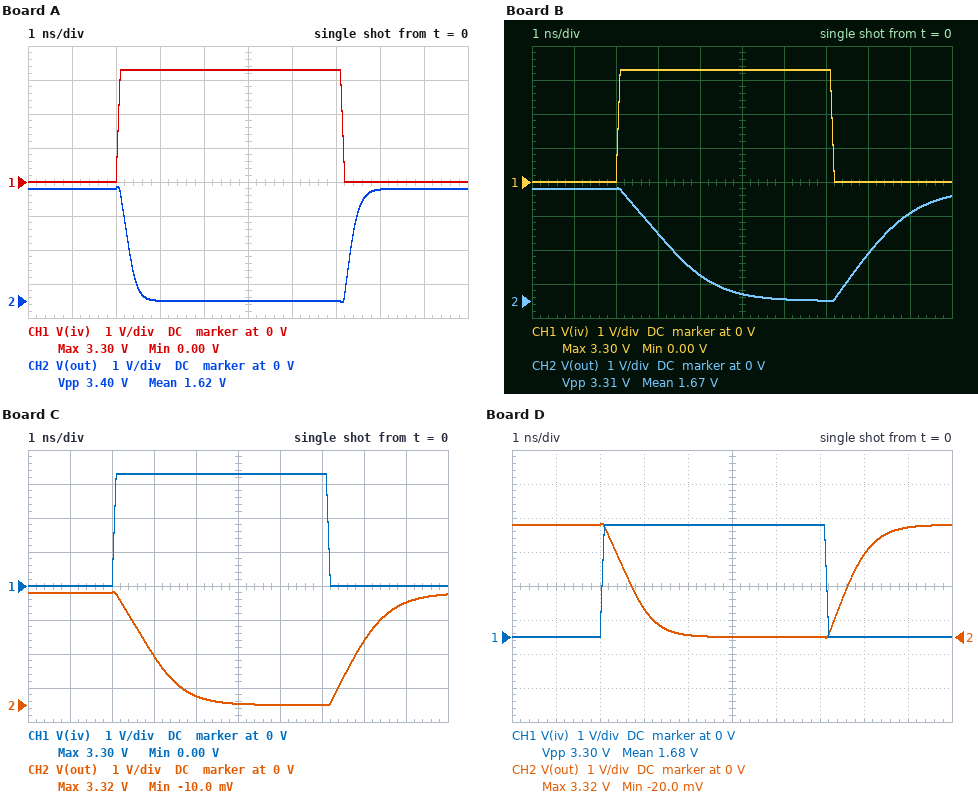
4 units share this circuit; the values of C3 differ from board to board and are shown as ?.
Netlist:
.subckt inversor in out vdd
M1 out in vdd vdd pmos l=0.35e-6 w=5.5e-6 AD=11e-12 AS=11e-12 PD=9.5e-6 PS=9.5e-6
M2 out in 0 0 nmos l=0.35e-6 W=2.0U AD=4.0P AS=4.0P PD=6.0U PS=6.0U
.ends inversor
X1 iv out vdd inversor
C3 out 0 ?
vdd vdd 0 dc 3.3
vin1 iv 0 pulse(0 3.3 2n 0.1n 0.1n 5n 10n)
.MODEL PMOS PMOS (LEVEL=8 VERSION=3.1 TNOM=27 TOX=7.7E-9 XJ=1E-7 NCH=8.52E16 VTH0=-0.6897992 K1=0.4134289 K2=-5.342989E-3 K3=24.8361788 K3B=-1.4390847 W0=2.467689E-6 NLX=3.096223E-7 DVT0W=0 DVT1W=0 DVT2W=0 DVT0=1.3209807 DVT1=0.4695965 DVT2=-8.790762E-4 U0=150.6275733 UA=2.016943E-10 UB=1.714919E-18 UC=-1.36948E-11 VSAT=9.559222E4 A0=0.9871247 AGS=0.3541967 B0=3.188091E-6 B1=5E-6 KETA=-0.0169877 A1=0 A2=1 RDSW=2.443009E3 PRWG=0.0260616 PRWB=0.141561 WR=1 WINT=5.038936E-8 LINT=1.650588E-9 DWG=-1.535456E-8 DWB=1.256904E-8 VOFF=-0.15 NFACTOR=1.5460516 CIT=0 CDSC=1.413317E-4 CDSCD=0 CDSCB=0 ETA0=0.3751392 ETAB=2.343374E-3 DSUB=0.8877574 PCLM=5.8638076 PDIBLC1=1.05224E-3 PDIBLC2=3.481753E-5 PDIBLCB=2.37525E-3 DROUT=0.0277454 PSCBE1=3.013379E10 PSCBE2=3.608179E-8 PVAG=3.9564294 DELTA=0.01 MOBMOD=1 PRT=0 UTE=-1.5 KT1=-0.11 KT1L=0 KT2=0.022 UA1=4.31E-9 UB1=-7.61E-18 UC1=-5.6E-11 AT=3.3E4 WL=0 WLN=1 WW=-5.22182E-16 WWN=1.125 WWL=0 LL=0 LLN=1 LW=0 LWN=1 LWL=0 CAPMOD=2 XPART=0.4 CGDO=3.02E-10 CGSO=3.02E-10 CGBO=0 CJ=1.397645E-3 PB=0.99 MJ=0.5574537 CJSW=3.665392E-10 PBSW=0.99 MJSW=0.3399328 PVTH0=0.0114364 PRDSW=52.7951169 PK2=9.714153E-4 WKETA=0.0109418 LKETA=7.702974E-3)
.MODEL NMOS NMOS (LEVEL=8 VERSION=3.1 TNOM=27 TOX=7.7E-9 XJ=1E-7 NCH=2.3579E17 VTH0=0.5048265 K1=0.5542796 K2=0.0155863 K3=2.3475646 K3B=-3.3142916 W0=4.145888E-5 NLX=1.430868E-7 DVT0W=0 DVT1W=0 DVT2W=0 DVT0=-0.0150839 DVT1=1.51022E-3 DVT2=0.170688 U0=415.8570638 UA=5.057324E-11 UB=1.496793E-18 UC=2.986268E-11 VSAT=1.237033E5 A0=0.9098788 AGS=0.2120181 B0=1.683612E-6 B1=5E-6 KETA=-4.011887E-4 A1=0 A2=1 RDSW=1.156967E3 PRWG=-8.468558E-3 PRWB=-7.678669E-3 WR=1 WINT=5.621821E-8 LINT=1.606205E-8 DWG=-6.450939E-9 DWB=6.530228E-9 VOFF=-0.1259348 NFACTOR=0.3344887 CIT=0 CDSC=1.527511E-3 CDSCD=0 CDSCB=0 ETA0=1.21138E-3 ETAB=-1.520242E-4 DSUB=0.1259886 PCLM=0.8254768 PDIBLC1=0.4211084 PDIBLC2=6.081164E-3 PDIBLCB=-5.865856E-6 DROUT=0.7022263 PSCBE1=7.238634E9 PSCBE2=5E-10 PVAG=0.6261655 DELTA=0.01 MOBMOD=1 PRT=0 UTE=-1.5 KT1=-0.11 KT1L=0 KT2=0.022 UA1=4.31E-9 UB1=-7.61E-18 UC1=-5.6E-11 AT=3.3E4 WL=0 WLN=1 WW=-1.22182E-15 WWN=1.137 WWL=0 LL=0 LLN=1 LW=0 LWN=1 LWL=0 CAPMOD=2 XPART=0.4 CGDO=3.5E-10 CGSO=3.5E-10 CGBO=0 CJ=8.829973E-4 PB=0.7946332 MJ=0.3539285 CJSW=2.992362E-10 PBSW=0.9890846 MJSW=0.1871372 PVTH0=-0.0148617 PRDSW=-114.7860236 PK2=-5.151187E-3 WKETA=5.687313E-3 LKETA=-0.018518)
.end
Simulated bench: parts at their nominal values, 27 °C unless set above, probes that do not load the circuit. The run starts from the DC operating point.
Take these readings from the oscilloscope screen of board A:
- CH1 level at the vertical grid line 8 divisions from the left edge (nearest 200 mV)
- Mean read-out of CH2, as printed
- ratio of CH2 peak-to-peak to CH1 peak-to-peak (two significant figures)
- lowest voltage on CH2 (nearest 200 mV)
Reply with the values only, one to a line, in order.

0 V
1.62 V
1.0
0 V
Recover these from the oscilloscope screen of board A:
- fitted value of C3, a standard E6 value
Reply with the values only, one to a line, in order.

100 fF
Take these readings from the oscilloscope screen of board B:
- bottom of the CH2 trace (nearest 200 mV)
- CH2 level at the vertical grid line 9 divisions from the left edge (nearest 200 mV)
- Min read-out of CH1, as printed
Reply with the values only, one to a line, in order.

0 V
2.6 V
0.00 V
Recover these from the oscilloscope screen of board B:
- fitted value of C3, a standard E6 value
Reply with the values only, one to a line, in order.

680 fF
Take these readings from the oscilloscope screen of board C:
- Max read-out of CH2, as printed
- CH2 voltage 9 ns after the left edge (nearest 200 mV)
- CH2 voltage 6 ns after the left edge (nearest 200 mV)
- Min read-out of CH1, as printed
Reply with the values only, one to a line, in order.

3.32 V
3.0 V
0 V
0.00 V
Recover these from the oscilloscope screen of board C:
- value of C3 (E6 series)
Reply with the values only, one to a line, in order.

470 fF
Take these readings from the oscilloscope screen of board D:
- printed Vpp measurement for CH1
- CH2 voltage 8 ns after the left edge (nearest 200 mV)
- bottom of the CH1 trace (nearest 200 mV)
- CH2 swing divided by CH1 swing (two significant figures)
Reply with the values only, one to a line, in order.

3.30 V
2.4 V
0 V
1.0
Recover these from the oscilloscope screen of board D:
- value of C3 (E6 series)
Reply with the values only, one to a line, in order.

330 fF
